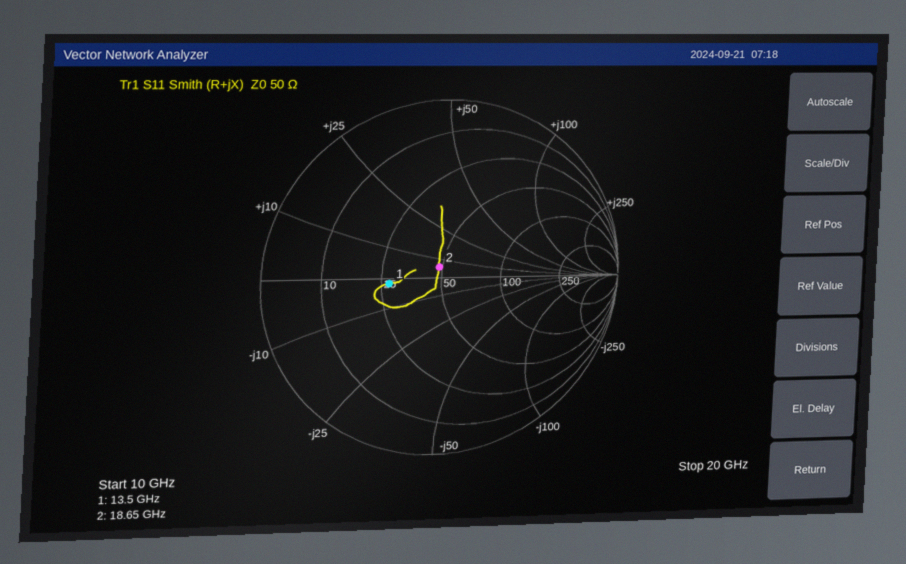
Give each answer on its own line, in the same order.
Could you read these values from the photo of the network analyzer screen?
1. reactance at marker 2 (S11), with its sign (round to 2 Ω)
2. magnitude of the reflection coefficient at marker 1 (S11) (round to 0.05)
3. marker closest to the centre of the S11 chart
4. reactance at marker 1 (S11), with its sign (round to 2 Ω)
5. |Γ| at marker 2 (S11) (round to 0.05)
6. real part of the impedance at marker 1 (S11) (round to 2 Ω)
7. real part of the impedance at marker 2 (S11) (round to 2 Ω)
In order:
+6 Ω
0.30
marker 2
-2 Ω
0.05
28 Ω
48 Ω
